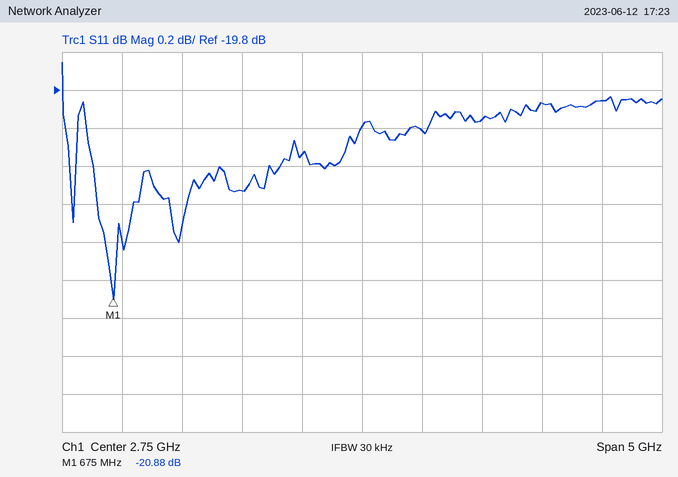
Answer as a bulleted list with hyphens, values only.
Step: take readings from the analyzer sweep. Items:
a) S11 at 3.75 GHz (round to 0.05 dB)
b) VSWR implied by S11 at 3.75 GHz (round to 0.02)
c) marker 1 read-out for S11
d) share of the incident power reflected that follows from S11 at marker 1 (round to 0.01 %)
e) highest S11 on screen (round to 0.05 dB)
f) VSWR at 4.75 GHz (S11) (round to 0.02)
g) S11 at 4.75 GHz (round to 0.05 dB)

- -19.95 dB
- 1.22
- -20.88 dB
- 0.82 %
- -19.65 dB
- 1.22
- -19.85 dB
